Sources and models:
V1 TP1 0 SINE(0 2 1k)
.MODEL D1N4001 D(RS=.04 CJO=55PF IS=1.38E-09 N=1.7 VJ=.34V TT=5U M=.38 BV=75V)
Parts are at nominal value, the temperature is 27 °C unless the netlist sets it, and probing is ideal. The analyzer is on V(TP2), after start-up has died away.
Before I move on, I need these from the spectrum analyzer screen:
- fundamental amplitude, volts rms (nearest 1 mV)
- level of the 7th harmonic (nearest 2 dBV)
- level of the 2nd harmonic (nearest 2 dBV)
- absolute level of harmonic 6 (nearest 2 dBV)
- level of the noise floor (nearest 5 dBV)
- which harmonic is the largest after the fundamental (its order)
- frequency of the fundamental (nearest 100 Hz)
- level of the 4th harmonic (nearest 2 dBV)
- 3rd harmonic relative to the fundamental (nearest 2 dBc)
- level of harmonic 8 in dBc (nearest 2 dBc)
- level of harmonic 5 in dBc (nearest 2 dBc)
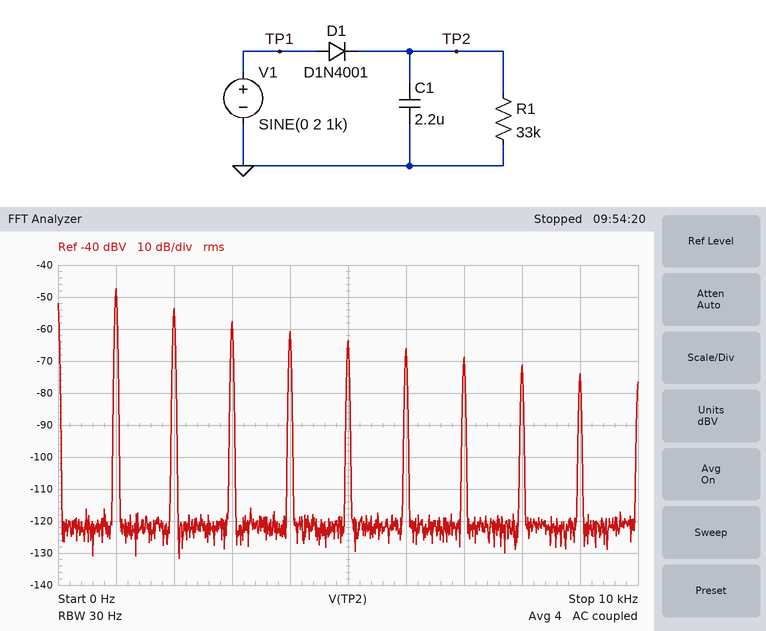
4 mV
-68 dBV
-54 dBV
-66 dBV
-120 dBV
2
1.0 kHz
-60 dBV
-10 dBc
-24 dBc
-16 dBc
